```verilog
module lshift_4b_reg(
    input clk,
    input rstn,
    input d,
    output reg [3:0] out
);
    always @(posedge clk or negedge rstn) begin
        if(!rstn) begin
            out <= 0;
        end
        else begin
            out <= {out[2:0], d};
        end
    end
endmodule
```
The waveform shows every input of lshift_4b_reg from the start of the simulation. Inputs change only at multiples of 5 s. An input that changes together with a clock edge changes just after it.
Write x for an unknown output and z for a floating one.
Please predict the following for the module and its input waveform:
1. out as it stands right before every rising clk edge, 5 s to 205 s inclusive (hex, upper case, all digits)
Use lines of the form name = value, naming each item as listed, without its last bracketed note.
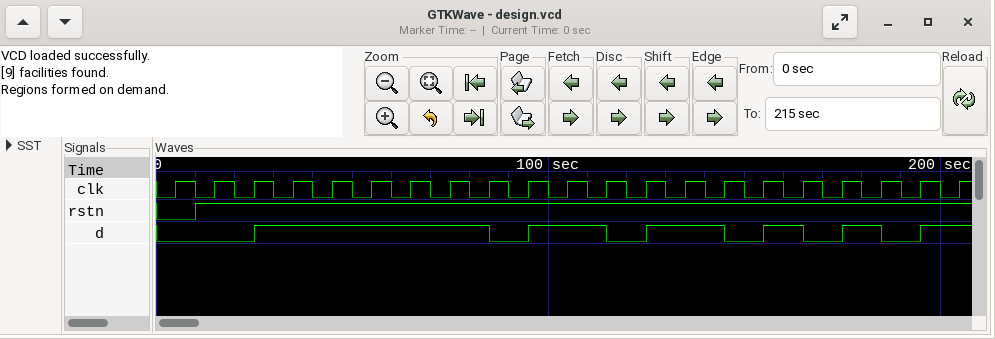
out as it stands right before every rising clk edge, 5 s to 205 s inclusive = 0, 0, 0, 0, 1, 3, 7, F, F, F, E, D, B, 6, D, B, 6, D, A, 5, A
